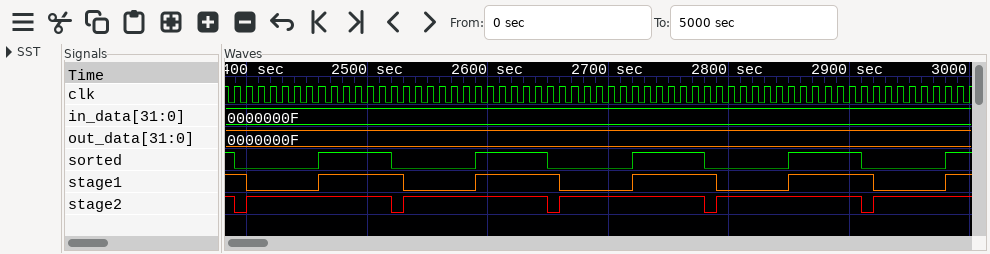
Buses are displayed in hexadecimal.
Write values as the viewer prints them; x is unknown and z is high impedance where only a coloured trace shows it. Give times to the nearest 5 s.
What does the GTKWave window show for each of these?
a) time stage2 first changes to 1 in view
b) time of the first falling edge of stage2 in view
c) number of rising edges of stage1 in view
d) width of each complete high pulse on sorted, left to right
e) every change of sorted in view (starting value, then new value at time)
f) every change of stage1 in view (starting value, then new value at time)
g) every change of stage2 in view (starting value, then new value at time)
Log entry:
2400 s
2390 s
5
60 s, 60 s, 60 s, 60 s
1, 0 at 2390 s, 1 at 2460 s, 0 at 2520 s, 1 at 2590 s, 0 at 2650 s, 1 at 2720 s, 0 at 2780 s, 1 at 2850 s, 0 at 2910 s, 1 at 2980 s
1, 0 at 2400 s, 1 at 2460 s, 0 at 2530 s, 1 at 2590 s, 0 at 2660 s, 1 at 2720 s, 0 at 2790 s, 1 at 2850 s, 0 at 2920 s, 1 at 2980 s
1, 0 at 2390 s, 1 at 2400 s, 0 at 2520 s, 1 at 2530 s, 0 at 2650 s, 1 at 2660 s, 0 at 2780 s, 1 at 2790 s, 0 at 2910 s, 1 at 2920 s
